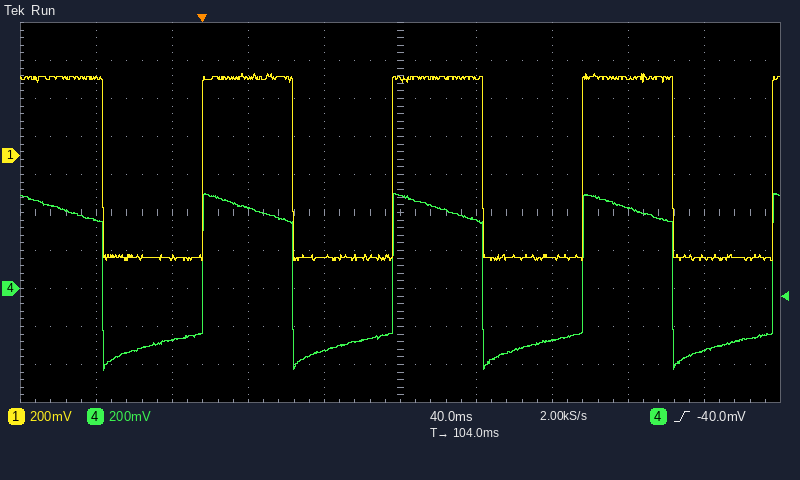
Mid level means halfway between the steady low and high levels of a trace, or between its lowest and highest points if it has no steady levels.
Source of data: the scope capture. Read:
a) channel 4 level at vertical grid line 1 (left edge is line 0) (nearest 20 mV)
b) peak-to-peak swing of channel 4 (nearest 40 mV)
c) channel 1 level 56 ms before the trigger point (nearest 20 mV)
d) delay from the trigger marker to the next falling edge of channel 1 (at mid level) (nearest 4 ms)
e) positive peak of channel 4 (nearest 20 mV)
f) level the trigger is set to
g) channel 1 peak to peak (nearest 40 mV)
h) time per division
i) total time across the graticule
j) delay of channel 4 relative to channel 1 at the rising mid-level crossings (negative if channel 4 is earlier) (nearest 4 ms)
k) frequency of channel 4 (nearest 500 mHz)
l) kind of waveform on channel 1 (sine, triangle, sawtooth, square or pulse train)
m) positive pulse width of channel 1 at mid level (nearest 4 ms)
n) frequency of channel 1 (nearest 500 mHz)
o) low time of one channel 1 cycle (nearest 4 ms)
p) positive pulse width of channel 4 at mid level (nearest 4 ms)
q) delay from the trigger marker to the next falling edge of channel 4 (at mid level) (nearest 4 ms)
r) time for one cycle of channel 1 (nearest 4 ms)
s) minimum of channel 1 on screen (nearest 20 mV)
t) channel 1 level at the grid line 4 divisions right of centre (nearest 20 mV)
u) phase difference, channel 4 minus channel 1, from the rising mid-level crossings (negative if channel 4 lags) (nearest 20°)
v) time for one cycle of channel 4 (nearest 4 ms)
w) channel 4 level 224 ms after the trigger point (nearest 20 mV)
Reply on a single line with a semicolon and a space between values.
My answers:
360 mV; 920 mV; 400 mV; 48 ms; 500 mV; -40.0 mV; 1.00 V; 40 ms; 400 ms; 0 ms; 10.0 Hz; square; 48 ms; 10.0 Hz; 52 ms; 48 ms; 48 ms; 100 ms; -560 mV; -540 mV; 0°; 100 ms; 420 mV
